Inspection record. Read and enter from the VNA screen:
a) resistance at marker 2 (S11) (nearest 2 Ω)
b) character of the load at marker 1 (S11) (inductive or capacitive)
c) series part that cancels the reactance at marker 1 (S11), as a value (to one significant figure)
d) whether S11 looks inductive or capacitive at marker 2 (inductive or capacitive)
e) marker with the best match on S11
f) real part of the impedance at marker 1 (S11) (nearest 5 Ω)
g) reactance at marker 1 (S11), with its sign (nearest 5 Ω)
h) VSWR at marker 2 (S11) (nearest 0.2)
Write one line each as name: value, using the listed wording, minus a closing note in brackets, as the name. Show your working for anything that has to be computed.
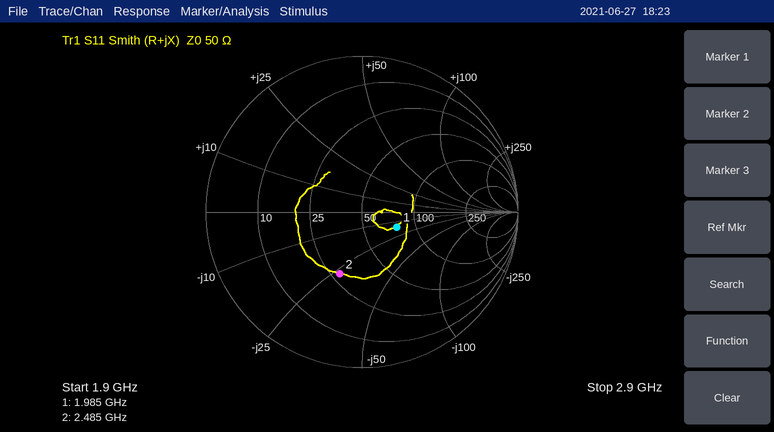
resistance at marker 2 (S11): 28 Ω
character of the load at marker 1 (S11): capacitive
series part that cancels the reactance at marker 1 (S11), as a value: L = 15 Ω/(2π × 1.985 GHz) ≈ 1 nH
whether S11 looks inductive or capacitive at marker 2: capacitive
marker with the best match on S11: marker 1
real part of the impedance at marker 1 (S11): 75 Ω
reactance at marker 1 (S11), with its sign: -15 Ω
VSWR at marker 2 (S11): 2.4
